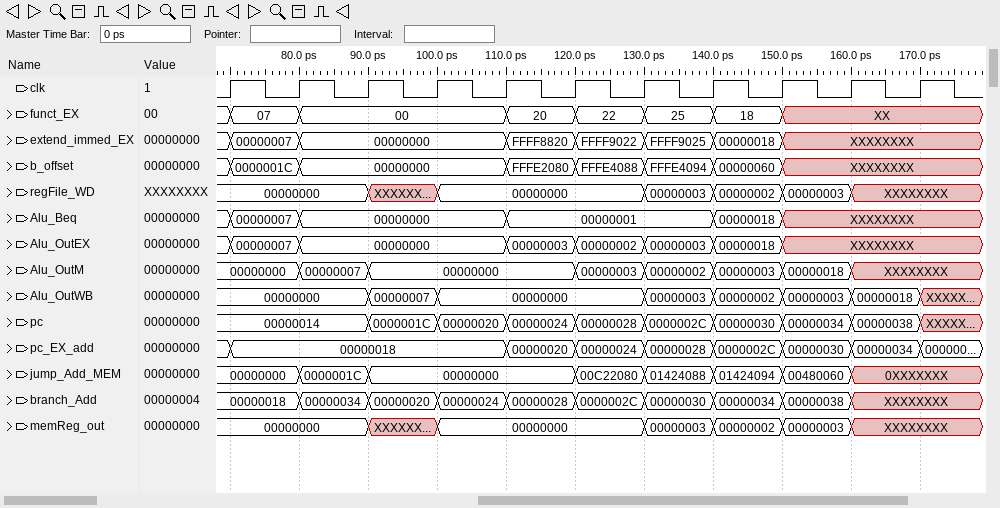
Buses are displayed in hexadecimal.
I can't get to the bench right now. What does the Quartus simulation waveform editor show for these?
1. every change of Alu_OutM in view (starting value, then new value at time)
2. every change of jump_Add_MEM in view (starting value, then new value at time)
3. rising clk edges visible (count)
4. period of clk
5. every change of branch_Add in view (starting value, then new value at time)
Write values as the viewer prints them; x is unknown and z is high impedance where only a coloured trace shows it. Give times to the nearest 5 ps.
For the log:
00000000, 00000007 at 80 ps, 00000000 at 90 ps, 00000003 at 120 ps, 00000002 at 130 ps, 00000003 at 140 ps, 00000018 at 150 ps, XXXXXXXX at 160 ps
00000000, 0000001C at 80 ps, 00000000 at 90 ps, 00C22080 at 120 ps, 01424088 at 130 ps, 01424094 at 140 ps, 00480060 at 150 ps, 0XXXXXXX at 160 ps
11
10 ps
00000018, 00000034 at 80 ps, 00000020 at 90 ps, 00000024 at 100 ps, 00000028 at 110 ps, 0000002C at 120 ps, 00000030 at 130 ps, 00000034 at 140 ps, 00000038 at 150 ps, XXXXXXXX at 160 ps
